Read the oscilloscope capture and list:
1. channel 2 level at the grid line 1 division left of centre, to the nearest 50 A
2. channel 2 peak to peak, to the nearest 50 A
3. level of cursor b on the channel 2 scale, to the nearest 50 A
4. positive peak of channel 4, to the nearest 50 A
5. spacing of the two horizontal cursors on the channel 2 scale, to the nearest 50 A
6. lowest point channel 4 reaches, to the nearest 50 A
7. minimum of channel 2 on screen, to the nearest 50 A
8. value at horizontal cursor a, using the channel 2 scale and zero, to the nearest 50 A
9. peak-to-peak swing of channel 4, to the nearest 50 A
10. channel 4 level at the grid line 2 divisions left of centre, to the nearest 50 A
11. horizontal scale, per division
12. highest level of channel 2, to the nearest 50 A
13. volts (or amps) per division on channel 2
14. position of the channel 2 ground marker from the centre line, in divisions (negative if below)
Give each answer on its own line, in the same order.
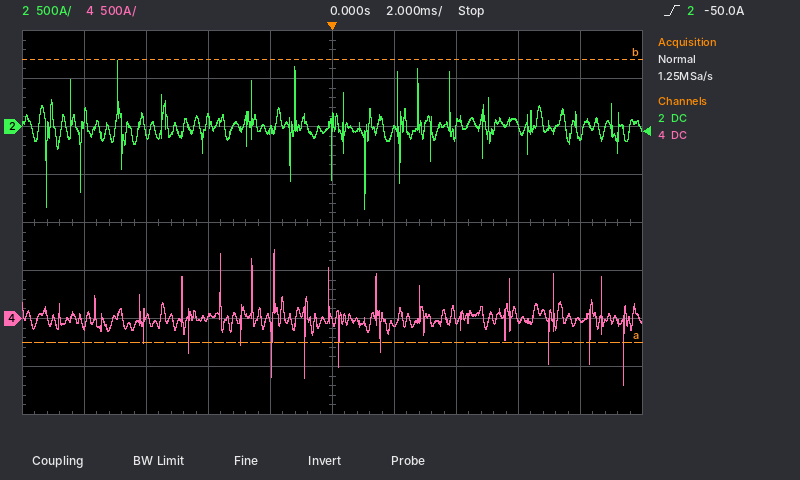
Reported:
-50 A
1.55 kA
700 A
700 A
2.95 kA
-700 A
-850 A
-2.25 kA
1.40 kA
0 A
2 ms
700 A
500 A
+2.0 div
